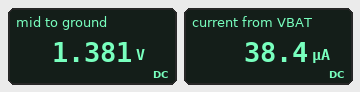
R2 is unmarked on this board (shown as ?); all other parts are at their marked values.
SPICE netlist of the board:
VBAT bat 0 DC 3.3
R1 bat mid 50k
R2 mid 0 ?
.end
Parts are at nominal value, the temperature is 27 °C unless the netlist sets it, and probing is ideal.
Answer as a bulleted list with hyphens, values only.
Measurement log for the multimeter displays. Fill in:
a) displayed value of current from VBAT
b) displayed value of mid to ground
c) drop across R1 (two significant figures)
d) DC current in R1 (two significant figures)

- 38.4 µA
- 1.381 V
- 1.9 V
- 38 µA
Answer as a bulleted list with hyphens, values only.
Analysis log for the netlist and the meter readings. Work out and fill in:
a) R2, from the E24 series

- 36 kΩ
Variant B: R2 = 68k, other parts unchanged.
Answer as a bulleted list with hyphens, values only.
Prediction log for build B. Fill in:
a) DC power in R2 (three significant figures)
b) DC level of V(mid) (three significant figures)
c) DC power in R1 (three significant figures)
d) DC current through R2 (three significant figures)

- 53.2 µW
- 1.90 V
- 39.1 µW
- 28.0 µA
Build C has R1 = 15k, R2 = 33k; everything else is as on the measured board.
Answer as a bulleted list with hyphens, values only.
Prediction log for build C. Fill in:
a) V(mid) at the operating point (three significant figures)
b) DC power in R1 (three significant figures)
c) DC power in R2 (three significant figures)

- 2.27 V
- 70.9 µW
- 156 µW
